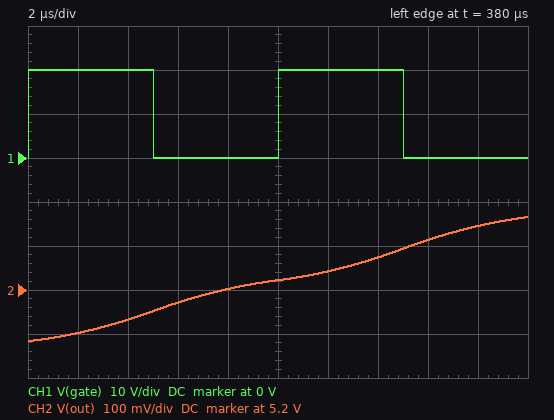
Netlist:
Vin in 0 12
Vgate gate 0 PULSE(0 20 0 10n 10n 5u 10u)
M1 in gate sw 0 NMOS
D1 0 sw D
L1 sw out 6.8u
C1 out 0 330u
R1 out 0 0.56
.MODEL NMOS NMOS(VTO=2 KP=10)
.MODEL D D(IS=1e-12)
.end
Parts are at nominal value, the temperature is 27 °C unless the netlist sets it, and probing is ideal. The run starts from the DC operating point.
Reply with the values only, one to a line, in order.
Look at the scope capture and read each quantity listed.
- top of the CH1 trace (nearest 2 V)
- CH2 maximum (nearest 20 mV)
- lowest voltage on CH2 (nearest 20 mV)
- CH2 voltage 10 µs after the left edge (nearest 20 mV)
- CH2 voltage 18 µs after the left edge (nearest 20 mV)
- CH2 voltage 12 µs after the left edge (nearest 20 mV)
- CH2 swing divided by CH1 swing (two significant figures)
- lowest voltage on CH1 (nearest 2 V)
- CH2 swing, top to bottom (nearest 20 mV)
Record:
20 V
5.36 V
5.08 V
5.22 V
5.34 V
5.24 V
0.014
0 V
280 mV
